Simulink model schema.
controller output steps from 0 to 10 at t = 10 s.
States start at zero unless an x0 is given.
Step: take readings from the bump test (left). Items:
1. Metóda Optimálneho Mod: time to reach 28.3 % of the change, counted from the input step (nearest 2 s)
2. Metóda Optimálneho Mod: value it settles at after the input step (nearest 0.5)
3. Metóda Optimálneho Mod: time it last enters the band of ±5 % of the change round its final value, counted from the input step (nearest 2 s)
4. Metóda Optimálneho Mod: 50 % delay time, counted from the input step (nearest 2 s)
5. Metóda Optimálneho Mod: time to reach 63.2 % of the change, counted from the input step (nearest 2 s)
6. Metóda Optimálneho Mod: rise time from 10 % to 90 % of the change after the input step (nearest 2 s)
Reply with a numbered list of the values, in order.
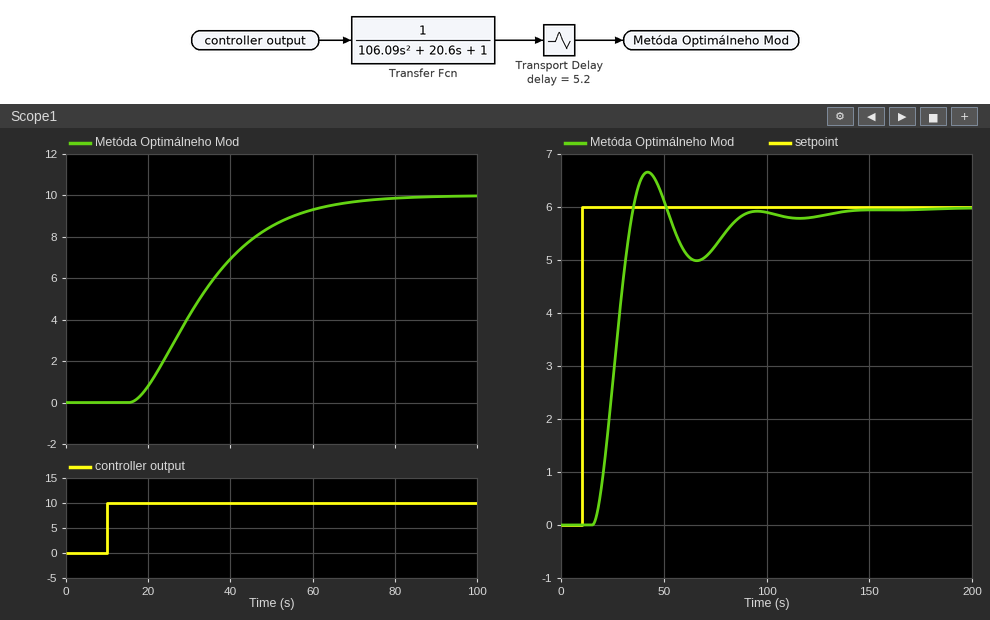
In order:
1. 16 s
2. 10.0
3. 54 s
4. 22 s
5. 28 s
6. 34 s
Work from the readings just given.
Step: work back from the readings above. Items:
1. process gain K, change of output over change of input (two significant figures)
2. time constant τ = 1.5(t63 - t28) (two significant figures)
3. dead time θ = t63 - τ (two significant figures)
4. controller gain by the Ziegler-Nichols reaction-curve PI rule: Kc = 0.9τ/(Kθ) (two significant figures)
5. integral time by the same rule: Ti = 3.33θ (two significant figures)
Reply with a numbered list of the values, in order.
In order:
1. 1.0
2. 18 s
3. 10 s
4. 1.6
5. 33 s
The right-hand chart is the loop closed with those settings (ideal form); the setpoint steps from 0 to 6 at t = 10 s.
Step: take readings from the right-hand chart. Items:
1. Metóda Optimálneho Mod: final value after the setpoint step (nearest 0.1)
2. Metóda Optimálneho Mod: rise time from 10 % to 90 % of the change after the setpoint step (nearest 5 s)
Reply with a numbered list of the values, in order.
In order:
1. 6.0
2. 15 s
